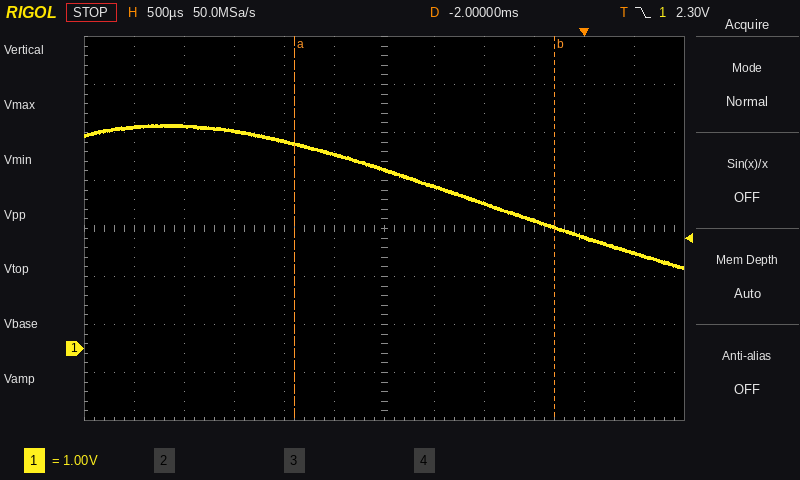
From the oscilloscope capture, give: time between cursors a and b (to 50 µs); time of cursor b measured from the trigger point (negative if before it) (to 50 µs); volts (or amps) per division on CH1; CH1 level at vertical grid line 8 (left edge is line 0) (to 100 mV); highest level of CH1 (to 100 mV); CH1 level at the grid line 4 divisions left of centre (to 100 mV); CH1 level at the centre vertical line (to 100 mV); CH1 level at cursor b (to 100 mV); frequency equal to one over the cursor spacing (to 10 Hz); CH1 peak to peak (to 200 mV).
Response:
2.60 ms
-300 µs
1 V
3.0 V
4.7 V
4.6 V
3.7 V
2.5 V
380 Hz
3.0 V
